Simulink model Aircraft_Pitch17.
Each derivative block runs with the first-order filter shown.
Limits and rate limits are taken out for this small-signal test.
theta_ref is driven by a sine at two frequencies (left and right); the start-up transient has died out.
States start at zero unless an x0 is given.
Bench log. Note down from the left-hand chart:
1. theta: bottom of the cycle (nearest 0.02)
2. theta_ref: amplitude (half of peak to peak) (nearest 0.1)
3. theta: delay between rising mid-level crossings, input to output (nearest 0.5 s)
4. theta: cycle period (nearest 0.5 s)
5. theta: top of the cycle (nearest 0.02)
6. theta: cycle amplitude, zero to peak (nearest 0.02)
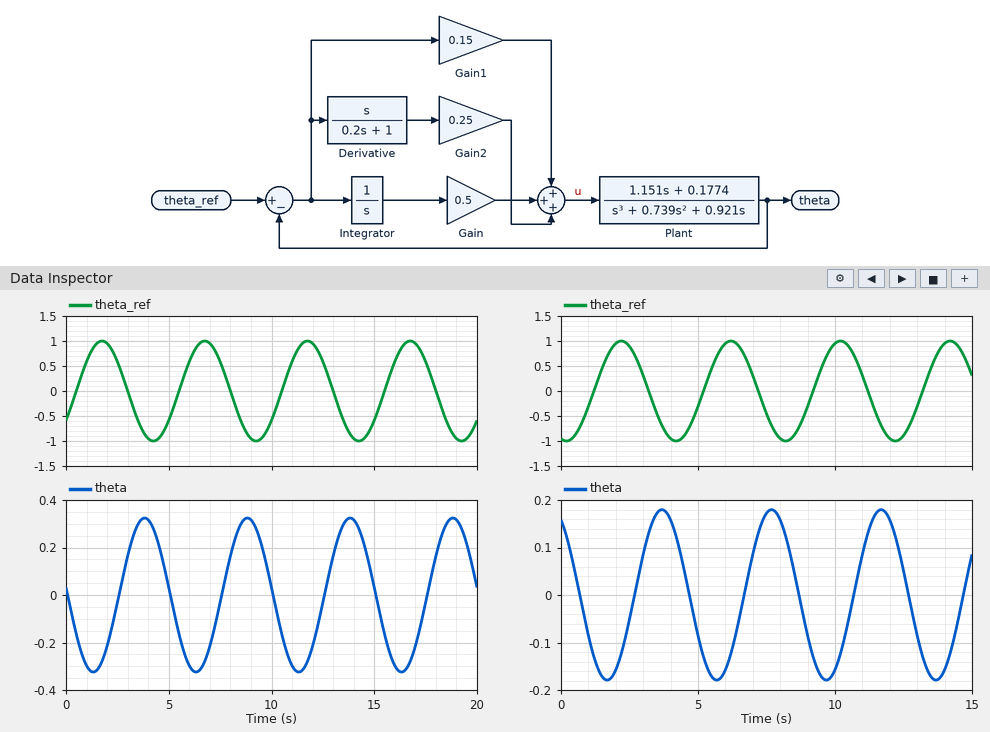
-0.32
1.0
2.0 s
5.0 s
0.32
0.32
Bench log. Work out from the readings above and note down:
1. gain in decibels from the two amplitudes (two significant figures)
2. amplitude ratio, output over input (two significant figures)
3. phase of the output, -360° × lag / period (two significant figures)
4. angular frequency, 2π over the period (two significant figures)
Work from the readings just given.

-9.9 dB
0.32
-140°
1.3 rad/s
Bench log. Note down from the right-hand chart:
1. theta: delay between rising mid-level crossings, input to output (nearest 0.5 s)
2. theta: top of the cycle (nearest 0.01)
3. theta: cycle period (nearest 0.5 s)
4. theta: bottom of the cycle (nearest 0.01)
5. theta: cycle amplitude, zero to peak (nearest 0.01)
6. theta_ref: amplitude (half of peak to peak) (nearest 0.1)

1.5 s
0.18
4.0 s
-0.18
0.18
1.0
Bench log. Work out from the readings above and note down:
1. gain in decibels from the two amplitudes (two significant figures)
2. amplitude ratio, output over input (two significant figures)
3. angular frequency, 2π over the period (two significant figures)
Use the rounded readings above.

-15 dB
0.18
1.6 rad/s
